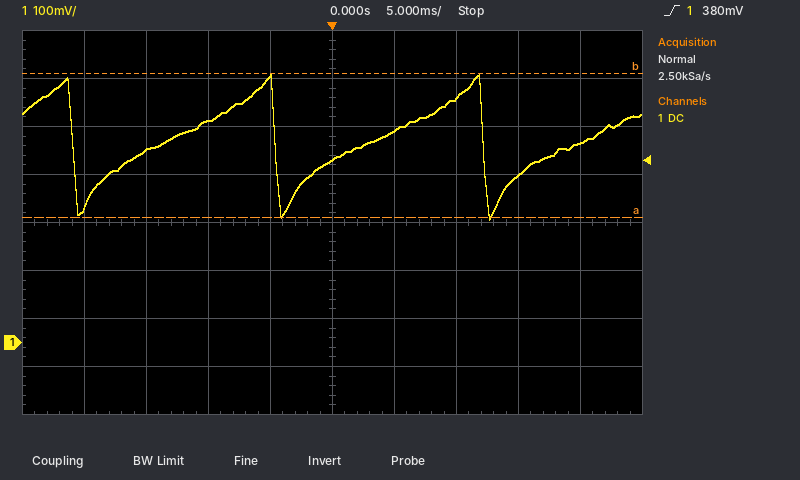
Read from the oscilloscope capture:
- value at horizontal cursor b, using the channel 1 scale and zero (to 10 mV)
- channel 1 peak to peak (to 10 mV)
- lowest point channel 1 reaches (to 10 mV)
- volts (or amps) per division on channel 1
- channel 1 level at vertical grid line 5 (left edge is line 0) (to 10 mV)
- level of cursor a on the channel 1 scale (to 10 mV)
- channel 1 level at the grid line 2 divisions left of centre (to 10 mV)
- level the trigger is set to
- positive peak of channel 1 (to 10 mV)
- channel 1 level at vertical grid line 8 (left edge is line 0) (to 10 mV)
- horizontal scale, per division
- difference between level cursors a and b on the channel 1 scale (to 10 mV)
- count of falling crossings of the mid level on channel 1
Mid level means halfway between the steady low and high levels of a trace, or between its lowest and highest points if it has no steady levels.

560 mV
300 mV
260 mV
100 mV
380 mV
260 mV
460 mV
380 mV
560 mV
350 mV
5 ms
300 mV
3
